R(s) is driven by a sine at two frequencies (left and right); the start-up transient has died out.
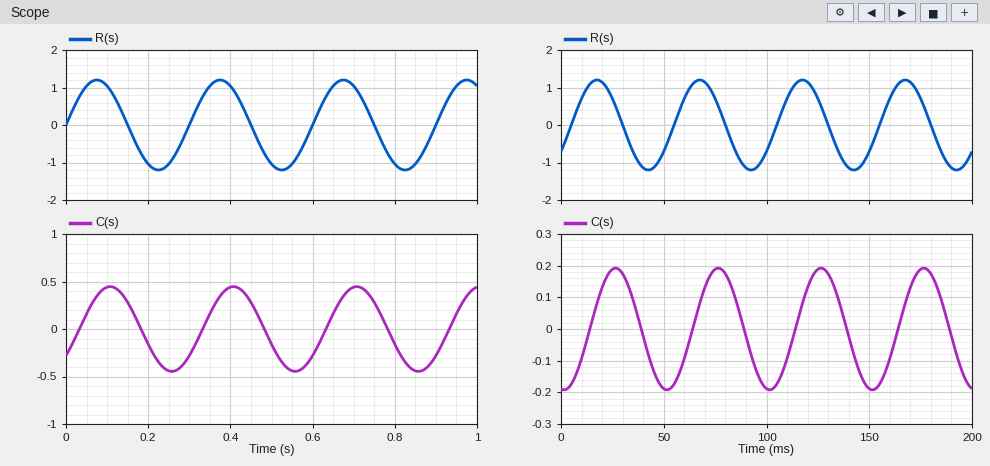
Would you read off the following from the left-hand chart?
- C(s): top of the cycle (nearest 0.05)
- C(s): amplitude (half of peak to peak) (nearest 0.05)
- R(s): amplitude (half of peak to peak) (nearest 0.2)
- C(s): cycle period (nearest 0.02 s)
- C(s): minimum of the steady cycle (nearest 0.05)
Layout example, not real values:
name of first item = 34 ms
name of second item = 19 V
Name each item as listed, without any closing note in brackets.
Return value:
C(s): top of the cycle = 0.45
C(s): amplitude (half of peak to peak) = 0.45
R(s): amplitude (half of peak to peak) = 1.2
C(s): cycle period = 0.30 s
C(s): minimum of the steady cycle = -0.45
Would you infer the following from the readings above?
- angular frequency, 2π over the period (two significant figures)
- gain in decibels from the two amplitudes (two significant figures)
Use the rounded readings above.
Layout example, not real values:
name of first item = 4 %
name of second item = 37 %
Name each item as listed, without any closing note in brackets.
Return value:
angular frequency, 2π over the period = 21 rad/s
gain in decibels from the two amplitudes = -8.5 dB
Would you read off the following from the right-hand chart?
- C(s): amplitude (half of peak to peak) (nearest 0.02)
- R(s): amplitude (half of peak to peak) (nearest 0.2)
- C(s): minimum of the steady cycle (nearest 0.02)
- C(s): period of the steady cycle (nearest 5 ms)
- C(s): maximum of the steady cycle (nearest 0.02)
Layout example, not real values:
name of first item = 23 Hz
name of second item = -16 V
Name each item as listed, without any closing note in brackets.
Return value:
C(s): amplitude (half of peak to peak) = 0.20
R(s): amplitude (half of peak to peak) = 1.2
C(s): minimum of the steady cycle = -0.20
C(s): period of the steady cycle = 50 ms
C(s): maximum of the steady cycle = 0.20
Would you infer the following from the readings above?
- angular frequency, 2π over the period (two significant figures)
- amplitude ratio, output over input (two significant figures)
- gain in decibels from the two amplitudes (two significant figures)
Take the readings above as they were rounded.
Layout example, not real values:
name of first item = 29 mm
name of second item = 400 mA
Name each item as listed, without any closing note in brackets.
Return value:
angular frequency, 2π over the period = 0.13 rad/ms
amplitude ratio, output over input = 0.17
gain in decibels from the two amplitudes = -16 dB
